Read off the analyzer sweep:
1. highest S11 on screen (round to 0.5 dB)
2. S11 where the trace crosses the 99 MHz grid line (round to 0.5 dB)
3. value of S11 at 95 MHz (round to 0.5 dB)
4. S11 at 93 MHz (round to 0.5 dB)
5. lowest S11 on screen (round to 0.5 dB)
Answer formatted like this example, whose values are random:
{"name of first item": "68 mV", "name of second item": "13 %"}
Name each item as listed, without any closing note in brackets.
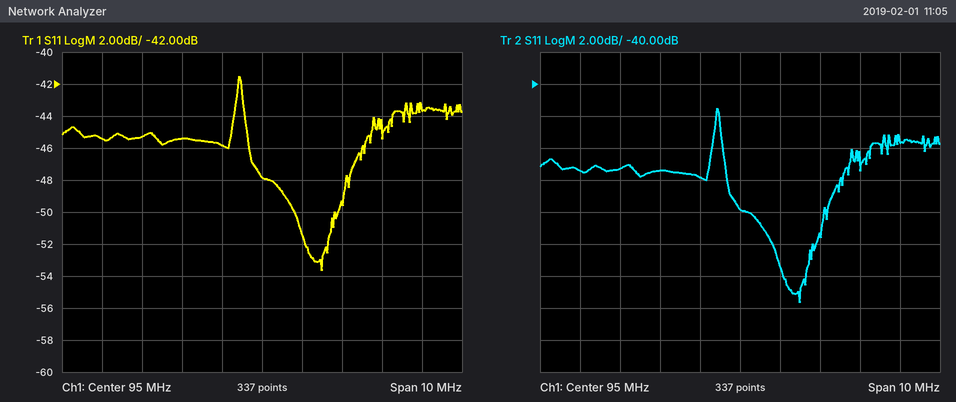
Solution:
{"highest S11 on screen": "-41.5 dB", "S11 where the trace crosses the 99 MHz grid line": "-43.5 dB", "value of S11 at 95 MHz": "-48.0 dB", "S11 at 93 MHz": "-45.5 dB", "lowest S11 on screen": "-53.5 dB"}
